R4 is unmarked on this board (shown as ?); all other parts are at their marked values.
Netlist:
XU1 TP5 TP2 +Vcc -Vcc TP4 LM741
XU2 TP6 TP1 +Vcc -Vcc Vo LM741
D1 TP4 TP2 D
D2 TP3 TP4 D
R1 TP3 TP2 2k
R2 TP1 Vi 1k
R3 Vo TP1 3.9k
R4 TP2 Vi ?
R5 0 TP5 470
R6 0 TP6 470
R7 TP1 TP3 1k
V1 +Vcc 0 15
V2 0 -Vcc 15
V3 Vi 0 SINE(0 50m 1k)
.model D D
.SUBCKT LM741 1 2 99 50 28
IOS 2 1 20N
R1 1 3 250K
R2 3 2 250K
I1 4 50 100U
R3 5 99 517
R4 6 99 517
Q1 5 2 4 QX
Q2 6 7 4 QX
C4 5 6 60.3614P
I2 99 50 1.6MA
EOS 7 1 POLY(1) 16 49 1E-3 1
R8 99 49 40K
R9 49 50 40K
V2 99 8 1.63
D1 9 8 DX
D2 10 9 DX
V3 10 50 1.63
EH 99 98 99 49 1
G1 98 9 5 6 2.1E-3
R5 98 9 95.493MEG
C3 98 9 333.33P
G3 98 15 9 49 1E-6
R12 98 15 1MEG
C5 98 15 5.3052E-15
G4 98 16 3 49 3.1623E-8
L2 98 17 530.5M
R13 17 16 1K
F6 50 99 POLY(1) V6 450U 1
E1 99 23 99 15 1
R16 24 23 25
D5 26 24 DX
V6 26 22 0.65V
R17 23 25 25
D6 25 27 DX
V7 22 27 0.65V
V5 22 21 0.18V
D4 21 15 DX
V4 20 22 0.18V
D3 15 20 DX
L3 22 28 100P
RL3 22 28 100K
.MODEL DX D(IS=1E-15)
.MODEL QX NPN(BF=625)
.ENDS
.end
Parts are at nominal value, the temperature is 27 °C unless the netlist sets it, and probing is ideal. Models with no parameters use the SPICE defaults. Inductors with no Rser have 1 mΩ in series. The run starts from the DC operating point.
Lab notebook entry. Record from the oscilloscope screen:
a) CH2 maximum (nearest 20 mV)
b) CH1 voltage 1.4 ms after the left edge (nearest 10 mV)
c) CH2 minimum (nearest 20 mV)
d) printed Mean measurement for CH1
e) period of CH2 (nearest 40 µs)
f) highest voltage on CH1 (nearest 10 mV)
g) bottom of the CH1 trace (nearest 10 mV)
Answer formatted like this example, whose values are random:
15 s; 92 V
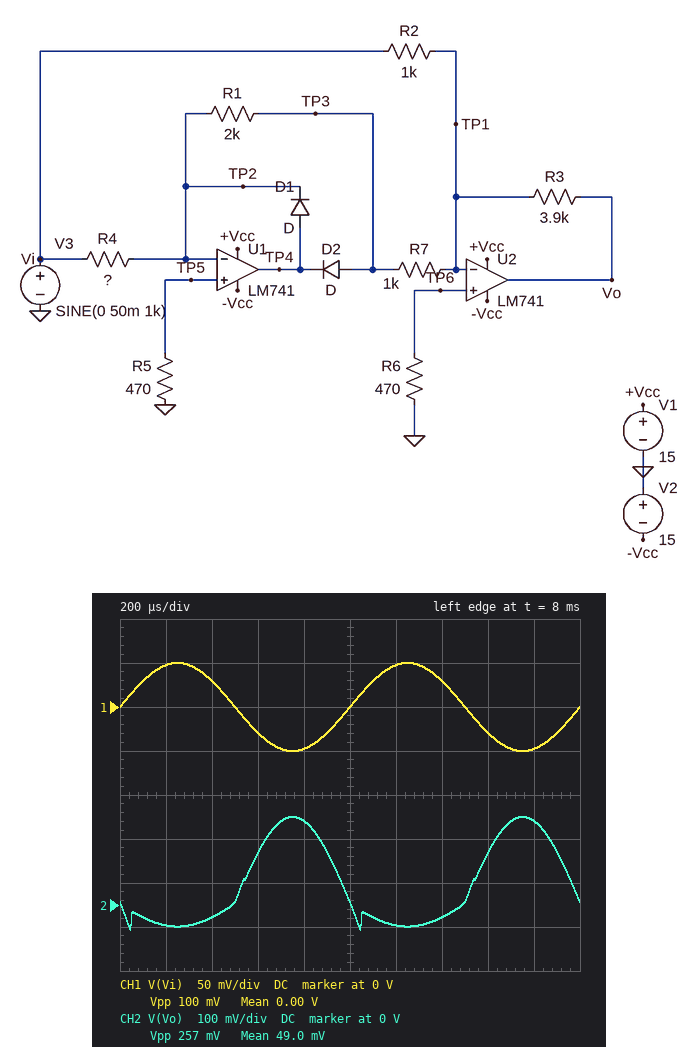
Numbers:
200 mV; 30 mV; -60 mV; 0.00 V; 1.00 ms; 50 mV; -50 mV
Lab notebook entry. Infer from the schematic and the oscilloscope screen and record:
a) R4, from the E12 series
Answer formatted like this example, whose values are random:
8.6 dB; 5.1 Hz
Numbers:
2.7 kΩ
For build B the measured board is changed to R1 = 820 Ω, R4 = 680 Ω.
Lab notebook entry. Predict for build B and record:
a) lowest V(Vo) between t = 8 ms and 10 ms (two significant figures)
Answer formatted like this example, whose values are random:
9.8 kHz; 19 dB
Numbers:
-58 mV
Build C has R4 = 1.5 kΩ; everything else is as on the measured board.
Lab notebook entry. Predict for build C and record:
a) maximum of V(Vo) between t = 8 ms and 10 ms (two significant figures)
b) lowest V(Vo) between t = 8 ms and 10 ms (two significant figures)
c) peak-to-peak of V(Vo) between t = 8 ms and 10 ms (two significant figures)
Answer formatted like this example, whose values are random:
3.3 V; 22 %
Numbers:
200 mV; -52 mV; 250 mV
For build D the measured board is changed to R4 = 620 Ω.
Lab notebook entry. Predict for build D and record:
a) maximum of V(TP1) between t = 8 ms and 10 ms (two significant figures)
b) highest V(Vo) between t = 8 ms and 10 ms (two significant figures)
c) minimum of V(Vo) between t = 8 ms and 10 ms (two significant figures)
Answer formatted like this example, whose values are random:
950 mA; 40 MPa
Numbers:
1.4 mV; 430 mV; -49 mV
